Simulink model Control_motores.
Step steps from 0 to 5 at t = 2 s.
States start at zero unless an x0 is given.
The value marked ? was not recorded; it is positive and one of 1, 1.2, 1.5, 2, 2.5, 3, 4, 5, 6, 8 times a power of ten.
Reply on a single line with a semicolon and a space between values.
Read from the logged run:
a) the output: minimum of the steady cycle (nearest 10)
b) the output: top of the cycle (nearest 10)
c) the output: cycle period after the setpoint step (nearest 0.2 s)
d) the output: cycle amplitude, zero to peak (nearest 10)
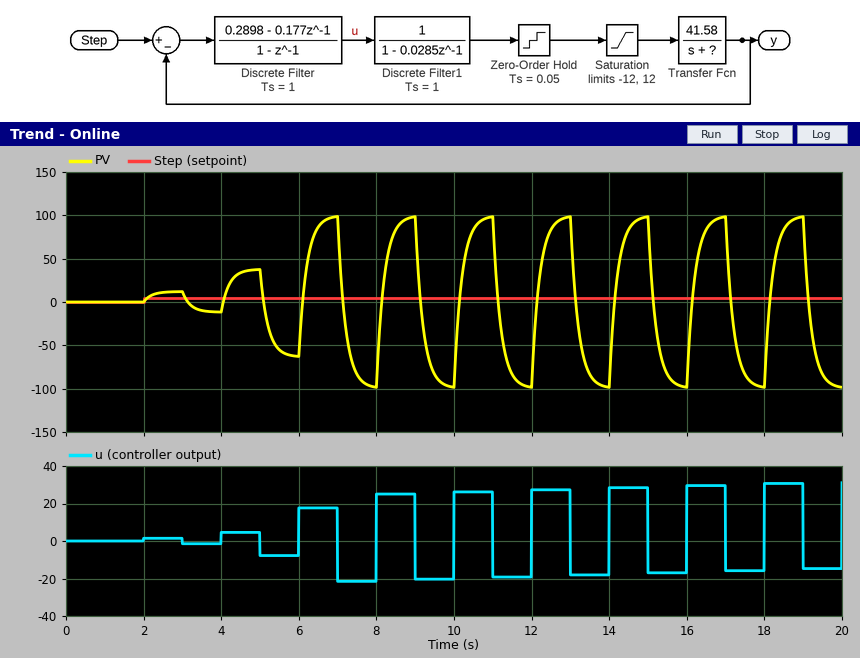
-100; 100; 2.0 s; 100
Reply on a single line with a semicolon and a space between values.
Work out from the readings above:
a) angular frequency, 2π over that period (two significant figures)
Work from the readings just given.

3.1 rad/s
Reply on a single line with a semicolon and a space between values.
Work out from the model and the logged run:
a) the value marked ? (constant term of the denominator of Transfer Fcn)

5
